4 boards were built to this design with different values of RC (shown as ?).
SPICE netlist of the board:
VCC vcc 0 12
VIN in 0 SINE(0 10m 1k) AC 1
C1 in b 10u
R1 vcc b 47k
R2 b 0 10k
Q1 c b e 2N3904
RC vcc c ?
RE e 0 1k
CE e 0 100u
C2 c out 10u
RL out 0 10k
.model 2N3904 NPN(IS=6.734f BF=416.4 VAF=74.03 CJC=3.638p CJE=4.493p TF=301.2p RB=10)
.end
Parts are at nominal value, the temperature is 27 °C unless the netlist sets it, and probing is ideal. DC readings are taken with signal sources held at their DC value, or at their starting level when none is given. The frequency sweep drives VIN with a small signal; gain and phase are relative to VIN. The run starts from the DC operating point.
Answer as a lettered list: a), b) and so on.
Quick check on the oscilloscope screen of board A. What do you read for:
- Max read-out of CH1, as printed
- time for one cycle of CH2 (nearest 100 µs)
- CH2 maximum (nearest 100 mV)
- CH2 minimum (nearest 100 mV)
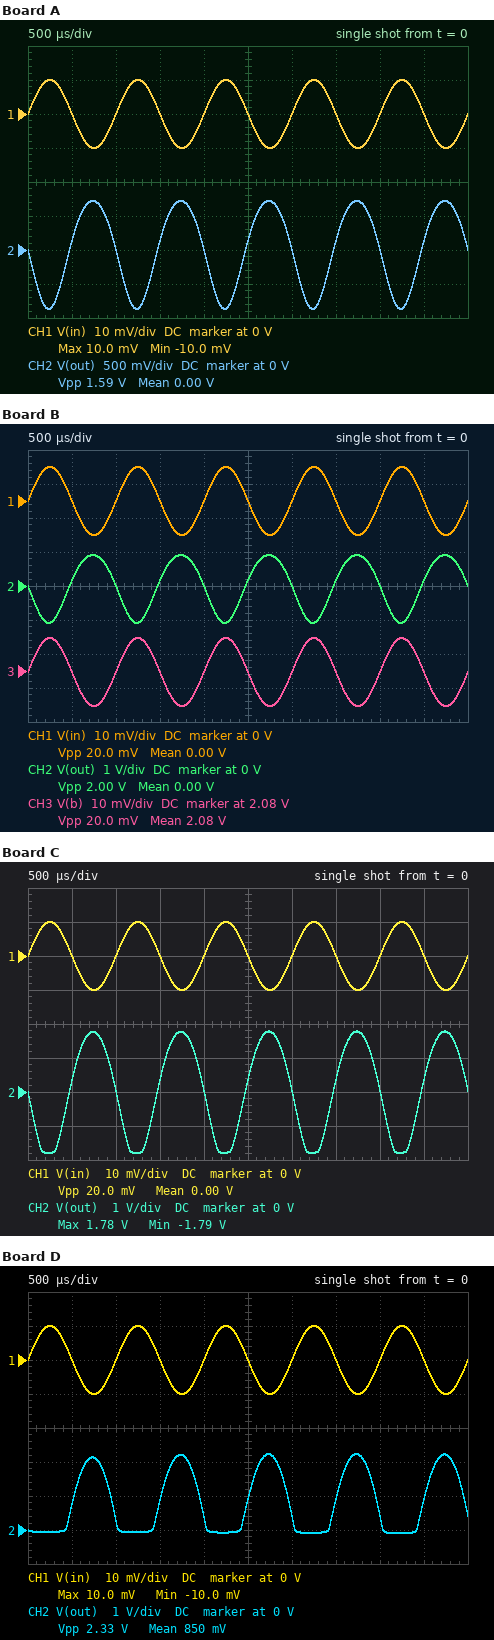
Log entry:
a) 10.0 mV
b) 1.0 ms
c) 700 mV
d) -900 mV
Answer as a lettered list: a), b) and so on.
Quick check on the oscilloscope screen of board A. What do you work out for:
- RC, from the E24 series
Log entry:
a) 1.8 kΩ
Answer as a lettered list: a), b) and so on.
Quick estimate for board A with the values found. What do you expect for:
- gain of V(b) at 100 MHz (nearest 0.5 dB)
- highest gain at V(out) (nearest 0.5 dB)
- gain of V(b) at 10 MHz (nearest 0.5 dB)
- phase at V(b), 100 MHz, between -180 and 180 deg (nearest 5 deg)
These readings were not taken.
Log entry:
a) 0 dB
b) 38.0 dB
c) 0 dB
d) 0 deg
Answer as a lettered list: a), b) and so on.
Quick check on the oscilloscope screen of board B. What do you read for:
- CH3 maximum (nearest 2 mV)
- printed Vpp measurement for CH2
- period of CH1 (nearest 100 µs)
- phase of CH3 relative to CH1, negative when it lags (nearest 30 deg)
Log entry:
a) 2.090 V
b) 2.00 V
c) 1.0 ms
d) 0 deg
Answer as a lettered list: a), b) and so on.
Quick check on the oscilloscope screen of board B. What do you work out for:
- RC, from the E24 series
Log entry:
a) 2.4 kΩ
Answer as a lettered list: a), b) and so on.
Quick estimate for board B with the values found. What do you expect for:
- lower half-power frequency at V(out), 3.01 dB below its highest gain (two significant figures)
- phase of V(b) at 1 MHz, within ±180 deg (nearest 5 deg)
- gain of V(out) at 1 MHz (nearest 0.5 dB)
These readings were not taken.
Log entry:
a) 87 Hz
b) 0 deg
c) 40.0 dB
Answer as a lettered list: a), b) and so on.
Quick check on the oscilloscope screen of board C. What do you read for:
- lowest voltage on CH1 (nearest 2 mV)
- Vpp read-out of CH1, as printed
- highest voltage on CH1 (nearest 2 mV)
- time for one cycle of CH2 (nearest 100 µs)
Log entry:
a) -10 mV
b) 20.0 mV
c) 10 mV
d) 1.0 ms
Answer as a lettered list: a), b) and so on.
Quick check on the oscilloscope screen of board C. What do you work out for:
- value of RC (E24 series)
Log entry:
a) 6.2 kΩ
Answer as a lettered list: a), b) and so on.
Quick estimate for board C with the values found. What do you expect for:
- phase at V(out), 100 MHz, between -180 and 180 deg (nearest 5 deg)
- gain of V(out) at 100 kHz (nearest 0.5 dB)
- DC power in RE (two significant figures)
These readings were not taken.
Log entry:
a) 90 deg
b) 45.5 dB
c) 2.0 mW
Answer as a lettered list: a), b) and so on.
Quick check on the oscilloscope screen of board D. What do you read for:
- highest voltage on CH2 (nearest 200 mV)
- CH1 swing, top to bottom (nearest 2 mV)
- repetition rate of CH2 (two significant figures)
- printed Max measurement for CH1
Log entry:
a) 2.2 V
b) 20 mV
c) 1.0 kHz
d) 10.0 mV
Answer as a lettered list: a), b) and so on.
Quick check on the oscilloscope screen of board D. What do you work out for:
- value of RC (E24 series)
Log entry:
a) 8.2 kΩ
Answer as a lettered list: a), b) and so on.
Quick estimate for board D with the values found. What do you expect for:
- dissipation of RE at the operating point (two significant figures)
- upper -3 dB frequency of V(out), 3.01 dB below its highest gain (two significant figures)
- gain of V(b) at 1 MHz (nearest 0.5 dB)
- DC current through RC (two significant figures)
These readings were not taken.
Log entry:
a) 1.7 mW
b) 28 MHz
c) 0 dB
d) 1.3 mA
